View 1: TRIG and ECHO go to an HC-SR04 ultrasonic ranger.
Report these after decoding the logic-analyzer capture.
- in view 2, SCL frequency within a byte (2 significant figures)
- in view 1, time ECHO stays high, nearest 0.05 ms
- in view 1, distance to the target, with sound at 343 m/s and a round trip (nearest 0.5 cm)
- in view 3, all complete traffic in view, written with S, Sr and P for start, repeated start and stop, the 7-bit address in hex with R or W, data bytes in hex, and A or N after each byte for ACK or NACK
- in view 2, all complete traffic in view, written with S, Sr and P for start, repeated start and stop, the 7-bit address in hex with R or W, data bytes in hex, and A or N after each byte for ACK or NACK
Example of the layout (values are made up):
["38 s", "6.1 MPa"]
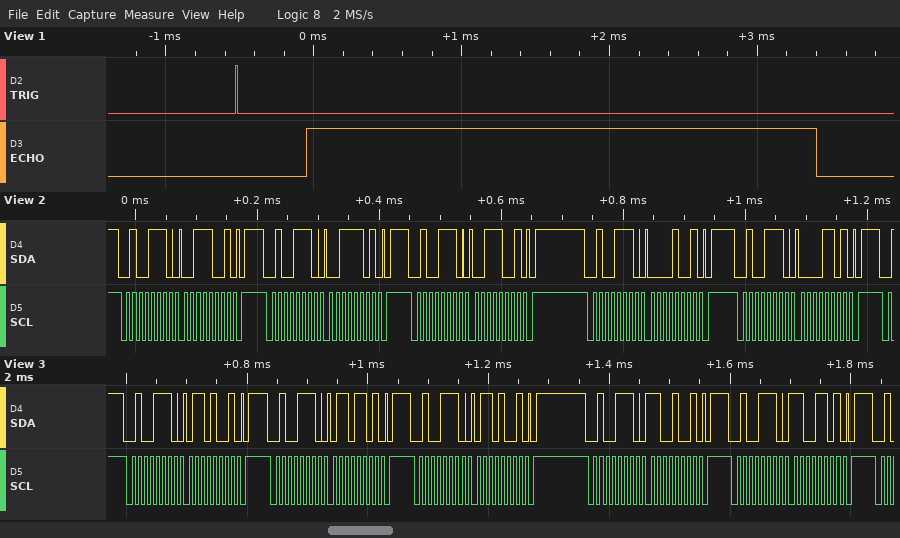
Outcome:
["100 kHz", "3.45 ms", "59 cm", "S 27W A 69 A P S 27W A 6D A P S 27W A 69 A P S 27W A C9 A P S 27W A CD A P", "S 27W A 39 A P S 27W A 3D A P S 27W A 39 A P S 27W A 09 A P S 27W A 0D A P"]
